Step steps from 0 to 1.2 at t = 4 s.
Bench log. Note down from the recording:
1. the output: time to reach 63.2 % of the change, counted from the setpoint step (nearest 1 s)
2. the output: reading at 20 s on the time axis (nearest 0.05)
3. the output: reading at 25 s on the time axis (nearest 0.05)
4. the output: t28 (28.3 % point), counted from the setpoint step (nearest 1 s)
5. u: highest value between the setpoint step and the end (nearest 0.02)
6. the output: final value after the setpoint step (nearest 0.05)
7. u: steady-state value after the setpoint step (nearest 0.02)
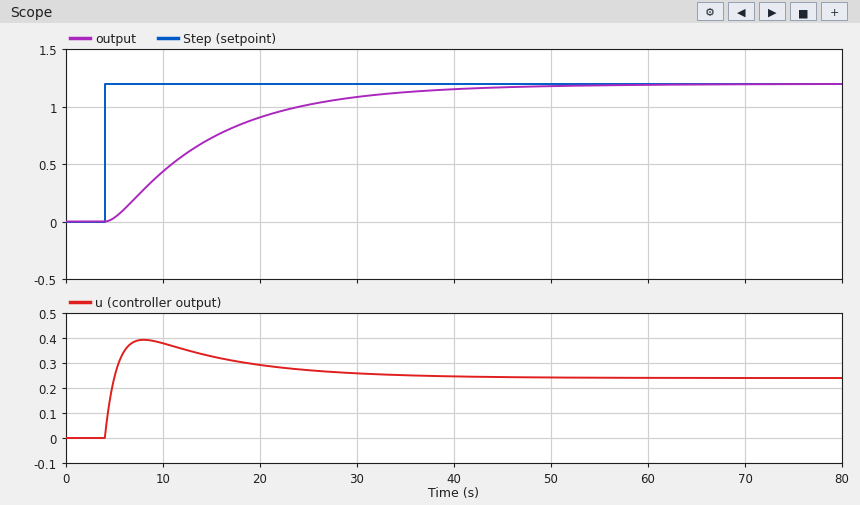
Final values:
12 s
0.90
1.00
5 s
0.40
1.20
0.24
